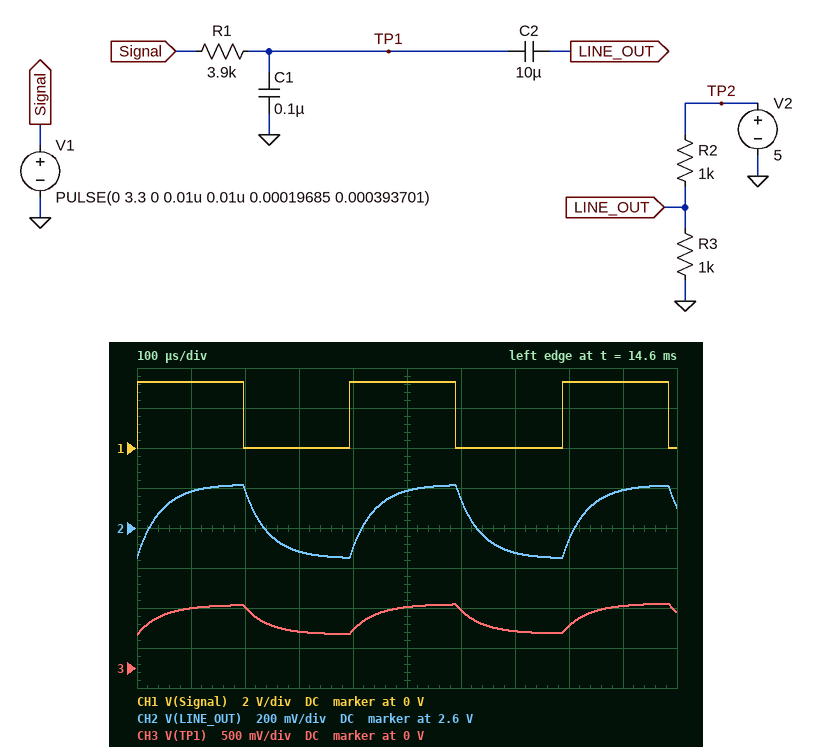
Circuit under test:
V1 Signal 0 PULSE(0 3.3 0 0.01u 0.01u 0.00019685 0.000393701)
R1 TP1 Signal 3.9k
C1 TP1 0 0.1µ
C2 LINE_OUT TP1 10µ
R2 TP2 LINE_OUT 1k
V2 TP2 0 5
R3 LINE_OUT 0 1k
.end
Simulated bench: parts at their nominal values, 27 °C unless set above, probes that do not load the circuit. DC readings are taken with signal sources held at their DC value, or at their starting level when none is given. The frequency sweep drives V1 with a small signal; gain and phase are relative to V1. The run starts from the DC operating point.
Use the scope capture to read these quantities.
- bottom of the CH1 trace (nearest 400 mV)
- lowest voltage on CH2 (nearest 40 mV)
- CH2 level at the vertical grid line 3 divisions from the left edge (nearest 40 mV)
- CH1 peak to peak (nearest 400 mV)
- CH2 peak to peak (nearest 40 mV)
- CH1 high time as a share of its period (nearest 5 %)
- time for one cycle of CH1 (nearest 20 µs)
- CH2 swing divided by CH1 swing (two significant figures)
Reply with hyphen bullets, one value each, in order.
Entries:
- 0 V
- 2.44 V
- 2.48 V
- 3.2 V
- 360 mV
- 50 %
- 400 µs
- 0.11
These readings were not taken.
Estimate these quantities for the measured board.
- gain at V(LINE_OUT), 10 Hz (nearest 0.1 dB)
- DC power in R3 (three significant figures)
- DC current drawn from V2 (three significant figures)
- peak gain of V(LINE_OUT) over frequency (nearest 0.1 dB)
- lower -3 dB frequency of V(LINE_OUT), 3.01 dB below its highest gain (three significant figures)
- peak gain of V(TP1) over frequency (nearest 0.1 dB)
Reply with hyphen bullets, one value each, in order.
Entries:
- -19.5 dB
- 6.25 mW
- 2.50 mA
- -19.0 dB
- 3.58 Hz
- 0 dB
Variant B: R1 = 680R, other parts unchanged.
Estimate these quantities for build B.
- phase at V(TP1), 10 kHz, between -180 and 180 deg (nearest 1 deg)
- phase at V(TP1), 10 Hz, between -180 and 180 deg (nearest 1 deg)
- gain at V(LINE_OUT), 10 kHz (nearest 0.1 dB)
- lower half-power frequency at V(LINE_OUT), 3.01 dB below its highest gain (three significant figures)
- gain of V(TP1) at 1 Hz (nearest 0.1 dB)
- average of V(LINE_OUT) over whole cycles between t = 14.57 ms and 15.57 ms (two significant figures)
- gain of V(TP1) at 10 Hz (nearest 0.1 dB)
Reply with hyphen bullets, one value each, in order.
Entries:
- -61 deg
- -19 deg
- -13.8 dB
- 13.4 Hz
- 0 dB
- 2.7 V
- -1.5 dB
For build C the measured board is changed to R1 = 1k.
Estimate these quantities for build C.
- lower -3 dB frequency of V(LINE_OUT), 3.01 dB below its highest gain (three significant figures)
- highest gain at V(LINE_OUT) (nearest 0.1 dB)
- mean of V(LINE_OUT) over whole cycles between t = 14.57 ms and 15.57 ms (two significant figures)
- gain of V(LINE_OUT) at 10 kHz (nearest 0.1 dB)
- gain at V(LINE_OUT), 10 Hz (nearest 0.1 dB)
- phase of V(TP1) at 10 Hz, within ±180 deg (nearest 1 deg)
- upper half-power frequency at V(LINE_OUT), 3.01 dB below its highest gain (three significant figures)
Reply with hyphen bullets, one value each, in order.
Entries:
- 10.5 Hz
- -9.6 dB
- 2.7 V
- -16.9 dB
- -12.8 dB
- -26 deg
- 4.82 kHz
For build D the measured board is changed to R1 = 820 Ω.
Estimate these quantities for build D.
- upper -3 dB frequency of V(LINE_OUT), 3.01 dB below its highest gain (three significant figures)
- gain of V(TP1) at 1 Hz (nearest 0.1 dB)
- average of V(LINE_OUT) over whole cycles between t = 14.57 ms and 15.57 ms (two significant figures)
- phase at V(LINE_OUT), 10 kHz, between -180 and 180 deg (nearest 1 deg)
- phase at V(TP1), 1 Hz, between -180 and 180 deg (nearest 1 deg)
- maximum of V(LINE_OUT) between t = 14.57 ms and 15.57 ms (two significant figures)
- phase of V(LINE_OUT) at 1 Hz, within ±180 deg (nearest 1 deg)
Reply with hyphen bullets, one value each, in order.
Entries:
- 5.17 kHz
- 0 dB
- 2.7 V
- -63 deg
- -3 deg
- 3.3 V
- 85 deg
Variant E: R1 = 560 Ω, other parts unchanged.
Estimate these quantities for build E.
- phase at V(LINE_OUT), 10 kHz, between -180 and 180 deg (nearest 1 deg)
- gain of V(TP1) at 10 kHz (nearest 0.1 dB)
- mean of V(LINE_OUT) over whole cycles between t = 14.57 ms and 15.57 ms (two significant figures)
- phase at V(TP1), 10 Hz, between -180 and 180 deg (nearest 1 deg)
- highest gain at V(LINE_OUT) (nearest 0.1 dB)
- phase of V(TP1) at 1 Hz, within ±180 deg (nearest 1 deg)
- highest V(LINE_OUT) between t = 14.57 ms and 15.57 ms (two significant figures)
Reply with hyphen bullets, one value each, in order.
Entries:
- -59 deg
- -12.3 dB
- 2.7 V
- -16 deg
- -6.6 dB
- -2 deg
- 3.5 V
